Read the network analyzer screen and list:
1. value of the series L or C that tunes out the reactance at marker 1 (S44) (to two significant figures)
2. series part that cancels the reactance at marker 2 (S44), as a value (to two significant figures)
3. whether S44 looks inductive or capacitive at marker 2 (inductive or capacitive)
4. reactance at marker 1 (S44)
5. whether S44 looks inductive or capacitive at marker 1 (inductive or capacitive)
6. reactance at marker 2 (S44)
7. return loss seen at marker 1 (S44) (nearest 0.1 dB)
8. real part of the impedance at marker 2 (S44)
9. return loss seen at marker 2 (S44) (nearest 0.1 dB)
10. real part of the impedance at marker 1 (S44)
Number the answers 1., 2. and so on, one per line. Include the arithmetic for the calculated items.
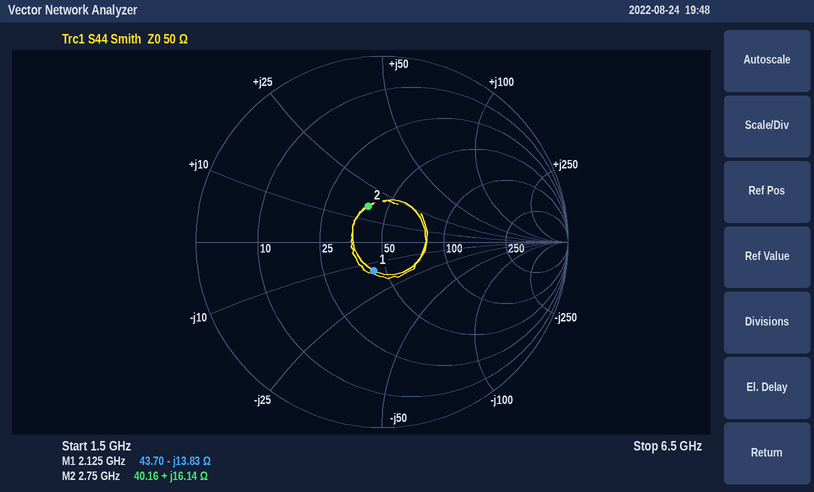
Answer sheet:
1. L = 13.83 Ω/(2π × 2.125 GHz) ≈ 1.0 nH
2. C = 1/(2π × 2.75 GHz × 16.14 Ω) ≈ 3.6 pF
3. inductive
4. -13.83 Ω
5. capacitive
6. +16.14 Ω
7. 15.9 dB
8. 40.16 Ω
9. 13.7 dB
10. 43.70 Ω
